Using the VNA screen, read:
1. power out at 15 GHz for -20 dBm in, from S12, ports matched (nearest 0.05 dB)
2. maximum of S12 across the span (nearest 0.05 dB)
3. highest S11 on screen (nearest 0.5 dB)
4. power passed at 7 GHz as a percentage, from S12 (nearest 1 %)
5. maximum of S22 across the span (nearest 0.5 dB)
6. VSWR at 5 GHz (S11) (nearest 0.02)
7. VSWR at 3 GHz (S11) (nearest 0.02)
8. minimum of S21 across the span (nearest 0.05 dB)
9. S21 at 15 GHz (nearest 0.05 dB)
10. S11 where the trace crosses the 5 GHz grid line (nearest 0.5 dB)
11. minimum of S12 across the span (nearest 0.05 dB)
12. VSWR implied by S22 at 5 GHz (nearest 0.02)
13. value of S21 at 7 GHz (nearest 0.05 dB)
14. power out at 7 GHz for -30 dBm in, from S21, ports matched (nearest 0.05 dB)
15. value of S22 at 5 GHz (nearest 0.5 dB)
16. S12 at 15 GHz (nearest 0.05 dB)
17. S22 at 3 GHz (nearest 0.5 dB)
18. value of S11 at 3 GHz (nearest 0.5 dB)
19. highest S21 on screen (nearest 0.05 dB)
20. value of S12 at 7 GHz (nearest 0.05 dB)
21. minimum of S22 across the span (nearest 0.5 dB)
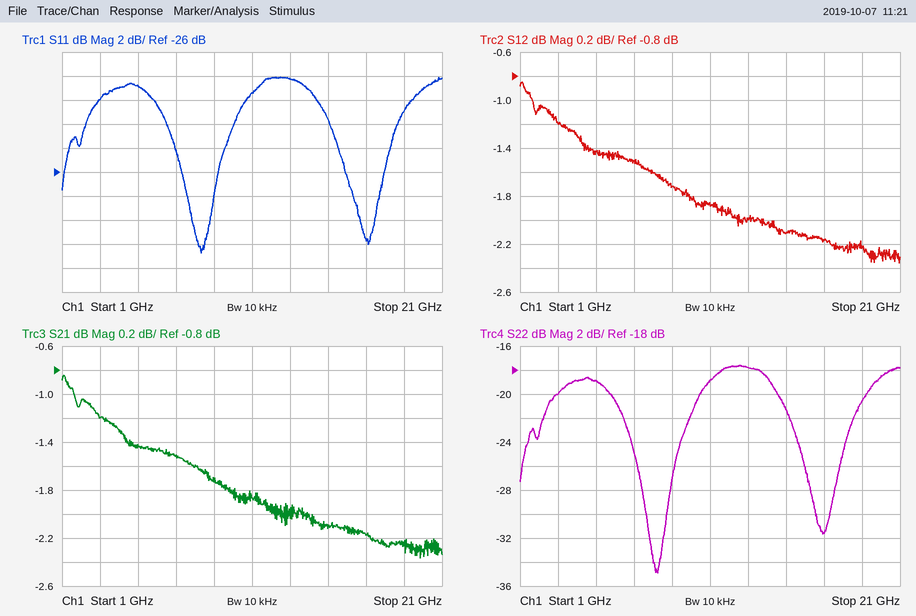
-22.10 dBm
-0.85 dB
-18.0 dB
71 %
-17.5 dB
1.26
1.22
-2.35 dB
-2.10 dB
-19.0 dB
-2.35 dB
1.26
-1.50 dB
-31.50 dBm
-19.0 dB
-2.10 dB
-20.0 dB
-20.0 dB
-0.85 dB
-1.50 dB
-35.0 dB
